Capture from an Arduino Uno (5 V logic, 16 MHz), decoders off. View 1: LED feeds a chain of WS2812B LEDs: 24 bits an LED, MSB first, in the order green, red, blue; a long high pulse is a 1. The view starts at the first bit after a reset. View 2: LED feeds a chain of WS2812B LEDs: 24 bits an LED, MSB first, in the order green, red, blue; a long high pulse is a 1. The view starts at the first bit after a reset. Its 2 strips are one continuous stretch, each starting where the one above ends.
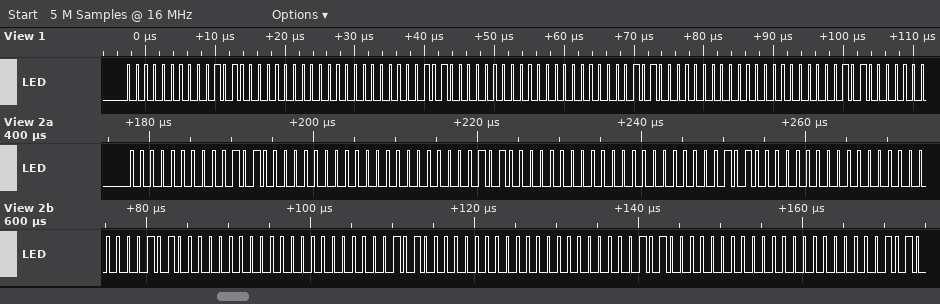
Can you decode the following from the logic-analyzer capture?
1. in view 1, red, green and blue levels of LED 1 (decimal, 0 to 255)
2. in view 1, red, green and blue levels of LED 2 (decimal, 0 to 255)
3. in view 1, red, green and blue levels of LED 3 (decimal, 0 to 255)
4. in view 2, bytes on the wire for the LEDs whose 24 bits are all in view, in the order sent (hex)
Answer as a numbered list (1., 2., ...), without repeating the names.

1. 40, 0, 0
2. 40, 0, 0
3. 40, 0, 0
4. 00 28 00 00 28 00 00 28 00 00 28 00 00 28 00 00 28 00
